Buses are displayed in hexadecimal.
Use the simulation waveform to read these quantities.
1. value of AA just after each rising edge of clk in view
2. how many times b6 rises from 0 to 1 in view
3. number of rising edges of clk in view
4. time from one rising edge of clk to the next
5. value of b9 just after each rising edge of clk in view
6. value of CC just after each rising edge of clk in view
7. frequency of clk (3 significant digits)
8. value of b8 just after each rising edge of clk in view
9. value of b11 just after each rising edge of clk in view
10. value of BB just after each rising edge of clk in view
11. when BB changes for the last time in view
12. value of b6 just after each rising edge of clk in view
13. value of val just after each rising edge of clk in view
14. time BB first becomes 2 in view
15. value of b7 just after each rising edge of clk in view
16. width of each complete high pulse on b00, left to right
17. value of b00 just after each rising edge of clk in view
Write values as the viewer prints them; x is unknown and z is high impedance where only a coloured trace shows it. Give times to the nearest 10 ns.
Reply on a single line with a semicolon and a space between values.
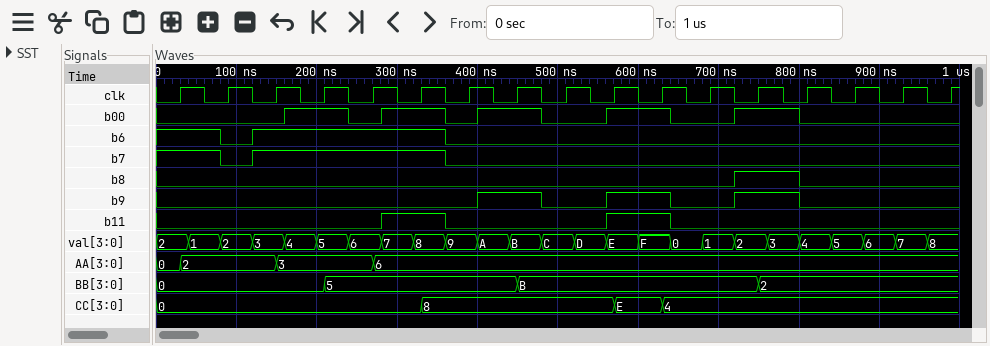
2, 2, 3, 3, 6, 6, 6, 6, 6, 6, 6, 6, 6, 6, 6, 6, 6; 1; 17; 60 ns; 0 0 0 0 0 0 0 1 0 1 1 0 1 0 0 0 0; 0, 0, 0, 0, 0, 8, 8, 8, 8, E, 4, 4, 4, 4, 4, 4, 4; 16.7 MHz; 0 0 0 0 0 0 0 0 0 0 0 0 1 0 0 0 0; 0 0 0 0 0 1 0 0 0 1 1 0 0 0 0 0 0; 0, 0, 0, 5, 5, 5, 5, B, B, B, B, B, 2, 2, 2, 2, 2; 750 ns; 1 0 1 1 1 1 0 0 0 0 0 0 0 0 0 0 0; 2, 2, 3, 5, 6, 8, 9, B, C, E, F, 1, 2, 4, 5, 7, 8; 750 ns; 1 0 1 1 1 1 0 0 0 0 0 0 0 0 0 0 0; 80 ns, 80 ns, 80 ns, 80 ns, 80 ns; 0 0 0 1 0 1 0 1 0 1 1 0 1 0 0 0 0
